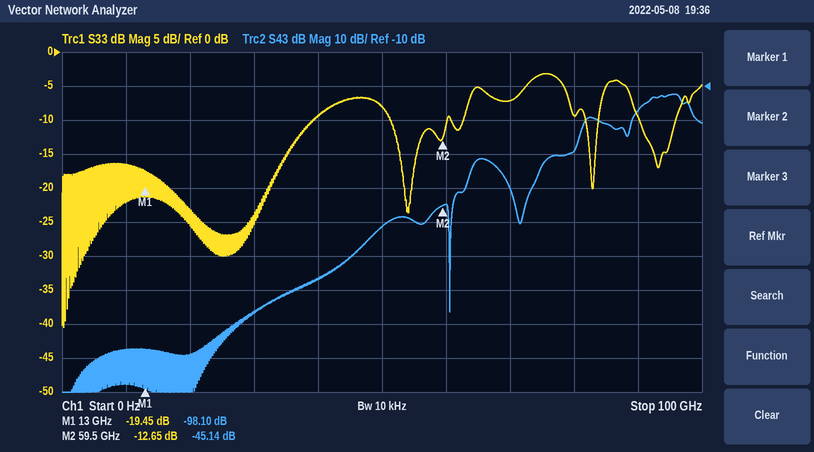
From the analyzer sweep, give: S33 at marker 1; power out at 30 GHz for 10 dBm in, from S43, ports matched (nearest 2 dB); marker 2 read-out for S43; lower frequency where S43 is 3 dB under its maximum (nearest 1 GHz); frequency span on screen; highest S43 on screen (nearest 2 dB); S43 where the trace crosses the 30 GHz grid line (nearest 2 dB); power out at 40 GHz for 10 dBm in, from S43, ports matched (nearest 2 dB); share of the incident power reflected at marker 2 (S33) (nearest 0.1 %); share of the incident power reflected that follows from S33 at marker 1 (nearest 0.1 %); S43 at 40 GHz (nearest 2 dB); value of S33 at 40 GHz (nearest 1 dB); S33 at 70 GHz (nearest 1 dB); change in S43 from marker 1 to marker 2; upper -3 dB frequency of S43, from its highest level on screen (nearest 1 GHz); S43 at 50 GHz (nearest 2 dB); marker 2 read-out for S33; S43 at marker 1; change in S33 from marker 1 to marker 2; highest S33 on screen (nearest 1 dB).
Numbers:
-19.45 dB
-66 dBm
-45.14 dB
91 GHz
100 GHz
-12 dB
-76 dB
-56 dBm
5.4 %
1.1 %
-66 dB
-9 dB
-7 dB
52.96 dB
98 GHz
-52 dB
-12.65 dB
-98.10 dB
6.80 dB
-3 dB
